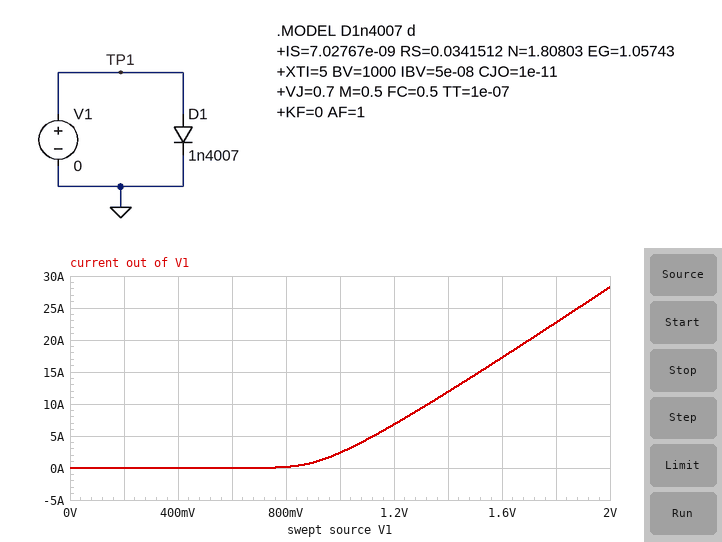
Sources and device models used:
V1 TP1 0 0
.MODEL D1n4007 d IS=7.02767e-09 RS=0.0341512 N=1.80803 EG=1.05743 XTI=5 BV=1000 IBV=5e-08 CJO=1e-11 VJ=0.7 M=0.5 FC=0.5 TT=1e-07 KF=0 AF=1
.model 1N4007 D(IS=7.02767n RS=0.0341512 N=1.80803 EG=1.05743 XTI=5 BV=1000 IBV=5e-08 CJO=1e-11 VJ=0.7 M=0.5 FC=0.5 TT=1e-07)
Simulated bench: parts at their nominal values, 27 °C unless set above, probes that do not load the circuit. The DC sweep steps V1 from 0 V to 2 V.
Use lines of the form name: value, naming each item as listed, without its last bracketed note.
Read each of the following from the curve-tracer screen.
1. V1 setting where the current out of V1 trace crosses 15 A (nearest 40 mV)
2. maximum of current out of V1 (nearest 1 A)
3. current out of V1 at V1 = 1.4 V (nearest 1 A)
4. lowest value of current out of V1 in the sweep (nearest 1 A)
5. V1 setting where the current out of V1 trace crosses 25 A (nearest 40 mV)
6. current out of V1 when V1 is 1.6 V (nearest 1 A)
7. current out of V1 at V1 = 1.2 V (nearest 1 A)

V1 setting where the current out of V1 trace crosses 15 A: 1.52 V
maximum of current out of V1: 28 A
current out of V1 at V1 = 1.4 V: 12 A
lowest value of current out of V1 in the sweep: 0 A
V1 setting where the current out of V1 trace crosses 25 A: 1.88 V
current out of V1 when V1 is 1.6 V: 17 A
current out of V1 at V1 = 1.2 V: 7 A
